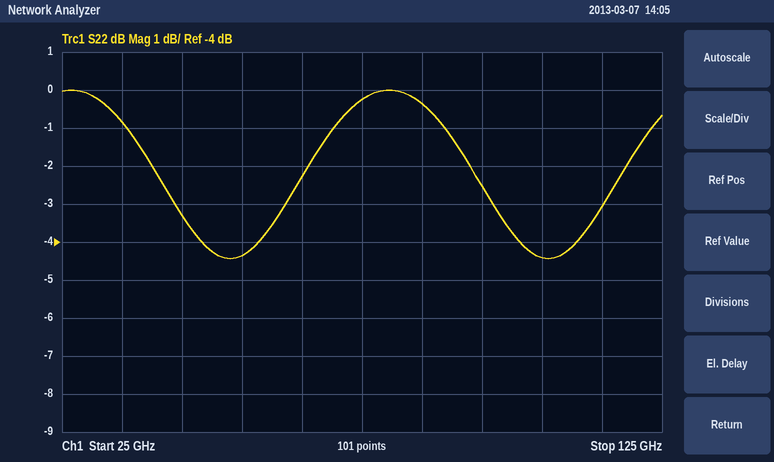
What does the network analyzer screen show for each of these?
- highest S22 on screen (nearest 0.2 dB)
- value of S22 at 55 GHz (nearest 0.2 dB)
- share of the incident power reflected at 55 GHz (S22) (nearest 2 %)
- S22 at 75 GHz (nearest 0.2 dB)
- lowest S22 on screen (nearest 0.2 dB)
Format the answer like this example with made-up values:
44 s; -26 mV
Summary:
0.0 dB; -4.4 dB; 36 %; -0.2 dB; -4.4 dB
